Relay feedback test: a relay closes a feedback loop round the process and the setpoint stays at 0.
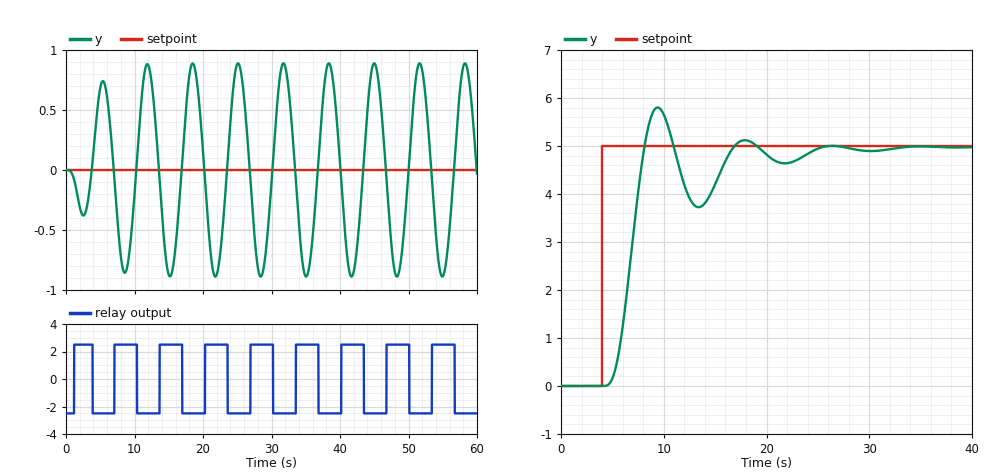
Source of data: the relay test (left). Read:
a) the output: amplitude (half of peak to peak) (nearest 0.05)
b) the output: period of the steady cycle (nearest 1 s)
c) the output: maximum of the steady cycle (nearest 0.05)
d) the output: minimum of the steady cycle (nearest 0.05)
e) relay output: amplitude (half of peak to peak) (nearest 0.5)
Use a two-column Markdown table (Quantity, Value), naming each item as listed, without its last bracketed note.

| Quantity | Value |
|---|---|
| the output: amplitude (half of peak to peak) | 0.90 |
| the output: period of the steady cycle | 7 s |
| the output: maximum of the steady cycle | 0.90 |
| the output: minimum of the steady cycle | -0.90 |
| relay output: amplitude (half of peak to peak) | 2.5 |
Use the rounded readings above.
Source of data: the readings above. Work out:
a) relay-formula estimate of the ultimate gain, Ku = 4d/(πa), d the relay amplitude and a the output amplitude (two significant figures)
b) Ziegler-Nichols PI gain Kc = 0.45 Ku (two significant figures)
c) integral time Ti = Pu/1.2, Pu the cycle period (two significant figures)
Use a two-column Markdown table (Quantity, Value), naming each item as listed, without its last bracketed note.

| Quantity | Value |
|---|---|
| relay-formula estimate of the ultimate gain, Ku = 4d/(πa), d the relay amplitude and a the output amplitude | 3.5 |
| Ziegler-Nichols PI gain Kc = 0.45 Ku | 1.6 |
| integral time Ti = Pu/1.2, Pu the cycle period | 5.8 s |
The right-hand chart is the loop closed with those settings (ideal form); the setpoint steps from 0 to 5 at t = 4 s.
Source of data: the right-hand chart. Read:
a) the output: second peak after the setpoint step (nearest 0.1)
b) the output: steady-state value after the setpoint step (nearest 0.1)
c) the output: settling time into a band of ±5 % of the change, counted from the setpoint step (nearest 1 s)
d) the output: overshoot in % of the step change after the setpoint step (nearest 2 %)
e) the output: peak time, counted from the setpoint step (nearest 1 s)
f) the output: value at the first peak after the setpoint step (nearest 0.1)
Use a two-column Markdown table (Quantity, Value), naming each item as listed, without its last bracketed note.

| Quantity | Value |
|---|---|
| the output: second peak after the setpoint step | 5.1 |
| the output: steady-state value after the setpoint step | 5.0 |
| the output: settling time into a band of ±5 % of the change, counted from the setpoint step | 19 s |
| the output: overshoot in % of the step change after the setpoint step | 16 % |
| the output: peak time, counted from the setpoint step | 5 s |
| the output: value at the first peak after the setpoint step | 5.8 |
